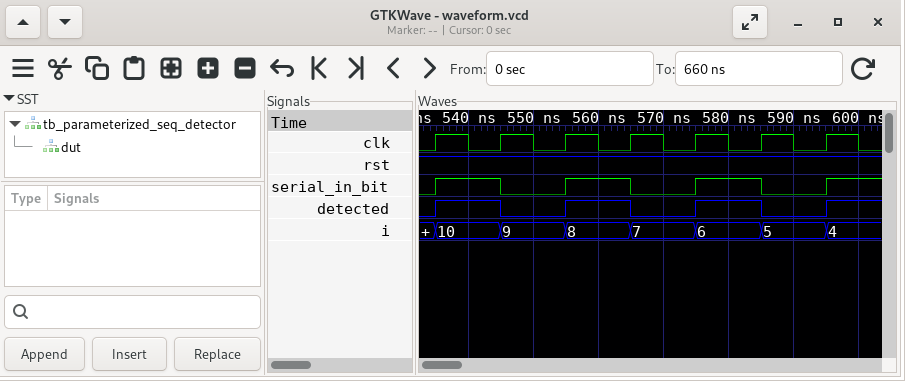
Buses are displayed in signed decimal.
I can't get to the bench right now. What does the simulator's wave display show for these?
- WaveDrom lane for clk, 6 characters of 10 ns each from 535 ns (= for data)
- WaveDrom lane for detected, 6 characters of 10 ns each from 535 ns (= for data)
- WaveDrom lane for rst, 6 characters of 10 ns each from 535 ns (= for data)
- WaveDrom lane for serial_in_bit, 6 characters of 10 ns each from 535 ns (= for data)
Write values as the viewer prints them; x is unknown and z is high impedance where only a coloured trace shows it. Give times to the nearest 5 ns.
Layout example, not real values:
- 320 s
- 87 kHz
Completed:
- {name: 'clk', wave: 'p.....'}
- {name: 'detected', wave: '101010'}
- {name: 'rst', wave: '1.....'}
- {name: 'serial_in_bit', wave: '101010'}
